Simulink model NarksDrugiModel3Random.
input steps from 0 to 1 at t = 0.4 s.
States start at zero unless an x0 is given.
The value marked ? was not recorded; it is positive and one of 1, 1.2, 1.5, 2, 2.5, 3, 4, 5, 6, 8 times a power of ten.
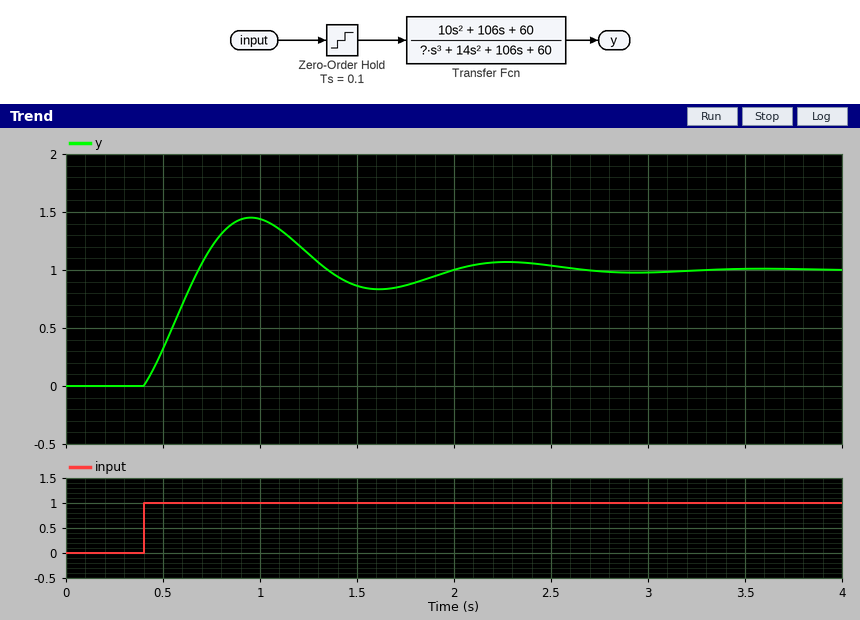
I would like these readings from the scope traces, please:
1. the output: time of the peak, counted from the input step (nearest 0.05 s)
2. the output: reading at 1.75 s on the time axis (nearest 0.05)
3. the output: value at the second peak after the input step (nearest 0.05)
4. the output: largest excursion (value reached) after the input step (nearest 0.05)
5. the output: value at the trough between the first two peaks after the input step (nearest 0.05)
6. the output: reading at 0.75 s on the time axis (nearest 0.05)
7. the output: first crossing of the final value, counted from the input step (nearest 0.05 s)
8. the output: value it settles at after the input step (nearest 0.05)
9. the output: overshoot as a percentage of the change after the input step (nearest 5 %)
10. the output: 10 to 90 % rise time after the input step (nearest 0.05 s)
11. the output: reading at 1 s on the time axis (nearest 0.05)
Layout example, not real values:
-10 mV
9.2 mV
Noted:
0.55 s
0.85
1.05
1.45
0.85
1.20
0.30 s
1.00
45 %
0.20 s
1.45
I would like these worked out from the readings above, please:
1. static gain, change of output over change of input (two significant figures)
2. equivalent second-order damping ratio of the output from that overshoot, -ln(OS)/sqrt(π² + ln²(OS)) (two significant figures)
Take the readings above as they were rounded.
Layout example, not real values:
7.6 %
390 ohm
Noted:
1.0
0.25
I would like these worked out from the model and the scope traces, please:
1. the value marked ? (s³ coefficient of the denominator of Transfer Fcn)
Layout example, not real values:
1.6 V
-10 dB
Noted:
4
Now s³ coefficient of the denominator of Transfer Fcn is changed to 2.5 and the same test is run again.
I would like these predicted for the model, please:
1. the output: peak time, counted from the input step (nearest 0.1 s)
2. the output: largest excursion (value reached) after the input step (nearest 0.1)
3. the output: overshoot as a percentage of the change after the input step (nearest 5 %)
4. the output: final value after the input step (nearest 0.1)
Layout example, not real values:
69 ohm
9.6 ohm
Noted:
0.4 s
1.3
35 %
1.0
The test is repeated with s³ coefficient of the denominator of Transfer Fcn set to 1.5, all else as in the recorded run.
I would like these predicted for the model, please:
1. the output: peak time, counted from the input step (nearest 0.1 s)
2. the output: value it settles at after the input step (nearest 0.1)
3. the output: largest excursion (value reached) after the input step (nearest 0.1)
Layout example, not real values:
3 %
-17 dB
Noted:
0.3 s
1.0
1.2
